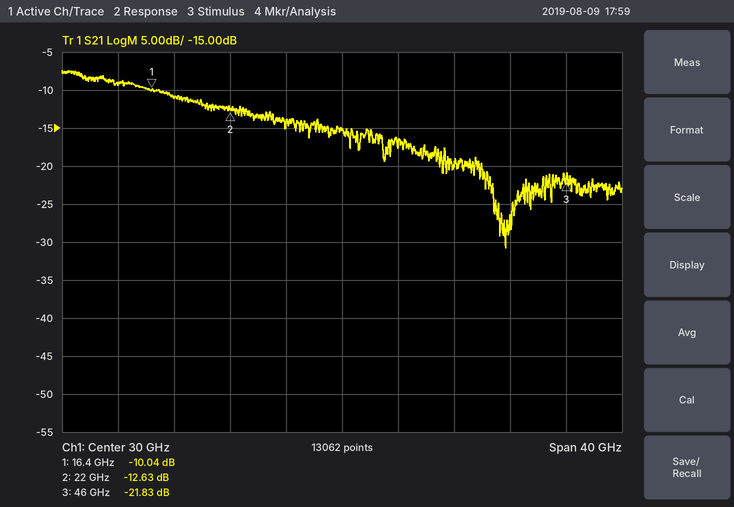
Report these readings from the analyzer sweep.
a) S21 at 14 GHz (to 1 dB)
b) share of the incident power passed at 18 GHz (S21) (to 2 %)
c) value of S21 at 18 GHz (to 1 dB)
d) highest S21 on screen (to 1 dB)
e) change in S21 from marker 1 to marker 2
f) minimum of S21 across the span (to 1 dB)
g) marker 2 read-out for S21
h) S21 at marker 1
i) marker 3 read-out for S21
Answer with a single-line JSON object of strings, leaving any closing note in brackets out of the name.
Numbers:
{"S21 at 14 GHz": "-9 dB", "share of the incident power passed at 18 GHz (S21)": "8 %", "value of S21 at 18 GHz": "-11 dB", "highest S21 on screen": "-7 dB", "change in S21 from marker 1 to marker 2": "-2.59 dB", "minimum of S21 across the span": "-31 dB", "marker 2 read-out for S21": "-12.63 dB", "S21 at marker 1": "-10.04 dB", "marker 3 read-out for S21": "-21.83 dB"}
